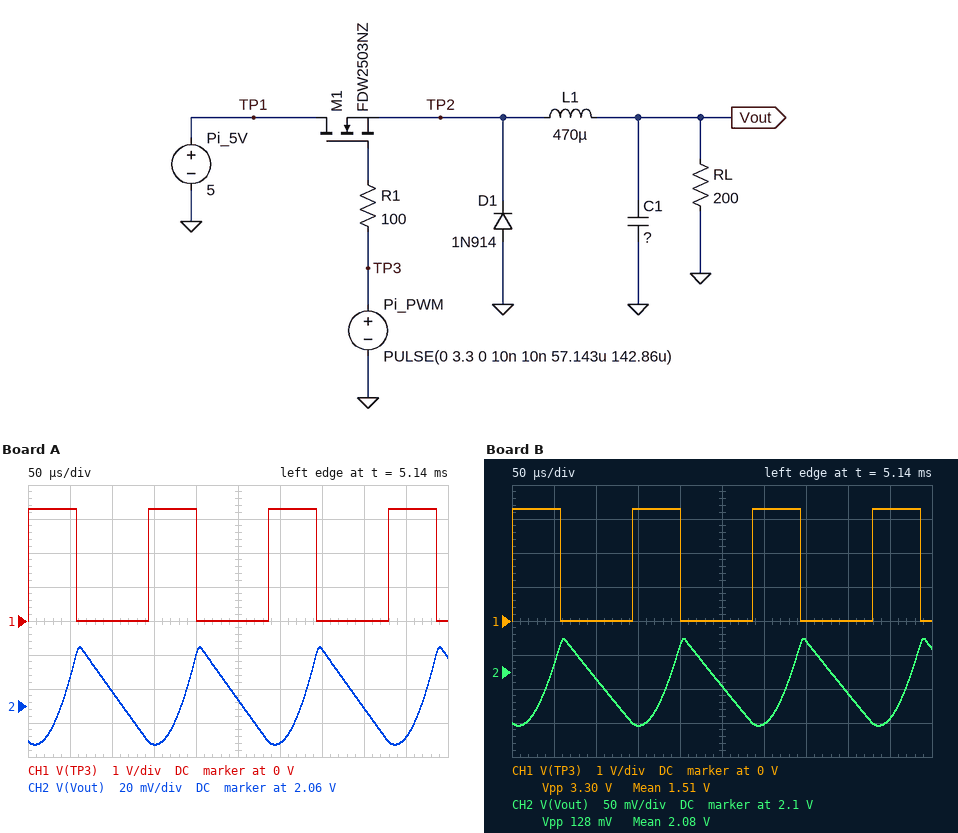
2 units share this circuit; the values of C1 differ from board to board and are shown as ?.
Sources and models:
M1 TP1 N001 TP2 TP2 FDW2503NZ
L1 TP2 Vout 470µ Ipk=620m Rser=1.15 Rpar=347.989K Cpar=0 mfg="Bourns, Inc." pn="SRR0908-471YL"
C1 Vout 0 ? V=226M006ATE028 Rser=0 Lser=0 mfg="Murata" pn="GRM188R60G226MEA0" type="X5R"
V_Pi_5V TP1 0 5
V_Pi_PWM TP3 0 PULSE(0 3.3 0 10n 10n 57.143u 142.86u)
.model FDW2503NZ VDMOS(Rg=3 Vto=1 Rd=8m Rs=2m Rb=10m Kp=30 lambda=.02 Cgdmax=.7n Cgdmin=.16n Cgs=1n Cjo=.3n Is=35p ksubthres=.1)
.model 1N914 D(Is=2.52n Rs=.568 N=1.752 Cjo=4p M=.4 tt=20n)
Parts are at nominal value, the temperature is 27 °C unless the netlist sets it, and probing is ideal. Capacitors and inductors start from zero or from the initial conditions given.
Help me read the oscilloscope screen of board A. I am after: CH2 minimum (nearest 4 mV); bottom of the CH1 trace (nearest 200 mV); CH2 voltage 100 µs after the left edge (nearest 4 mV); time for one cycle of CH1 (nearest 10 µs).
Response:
2.036 V
0 V
2.068 V
140 µs
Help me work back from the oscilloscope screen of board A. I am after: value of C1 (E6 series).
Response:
15 µF
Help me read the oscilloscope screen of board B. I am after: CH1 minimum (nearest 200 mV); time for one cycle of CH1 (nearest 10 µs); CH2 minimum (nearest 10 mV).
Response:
0 V
140 µs
2.02 V
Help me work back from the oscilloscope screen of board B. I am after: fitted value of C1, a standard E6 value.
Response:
6.8 µF
